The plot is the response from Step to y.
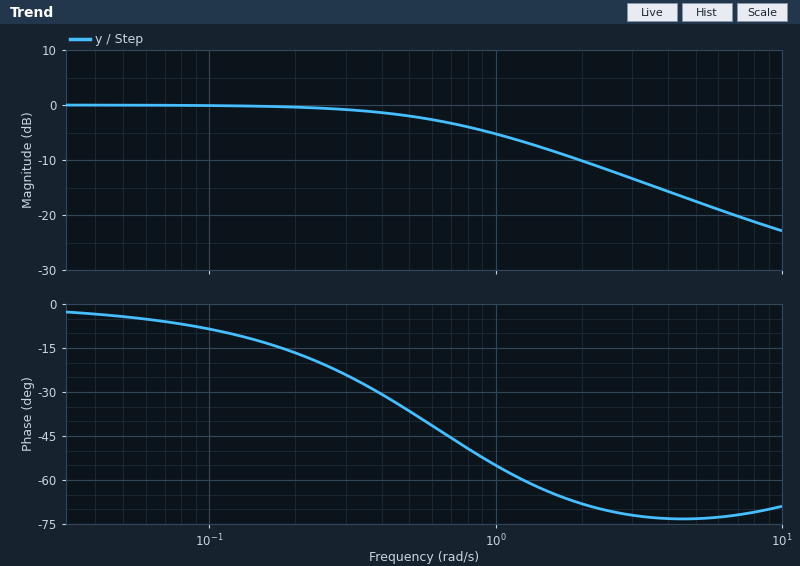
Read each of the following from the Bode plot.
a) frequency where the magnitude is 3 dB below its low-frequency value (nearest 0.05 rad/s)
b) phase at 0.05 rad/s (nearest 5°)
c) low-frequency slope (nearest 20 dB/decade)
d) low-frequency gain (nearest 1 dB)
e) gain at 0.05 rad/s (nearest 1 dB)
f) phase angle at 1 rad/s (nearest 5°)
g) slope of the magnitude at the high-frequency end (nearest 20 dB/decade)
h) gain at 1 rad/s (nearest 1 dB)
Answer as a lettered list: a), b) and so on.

a) 0.65 rad/s
b) -5°
c) 0 dB/decade
d) 0 dB
e) 0 dB
f) -55°
g) -20 dB/decade
h) -5 dB
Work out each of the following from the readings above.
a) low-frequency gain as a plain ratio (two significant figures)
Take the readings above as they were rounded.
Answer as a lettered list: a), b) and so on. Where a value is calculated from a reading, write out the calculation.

a) 10^(0 / 20) = 1.0
